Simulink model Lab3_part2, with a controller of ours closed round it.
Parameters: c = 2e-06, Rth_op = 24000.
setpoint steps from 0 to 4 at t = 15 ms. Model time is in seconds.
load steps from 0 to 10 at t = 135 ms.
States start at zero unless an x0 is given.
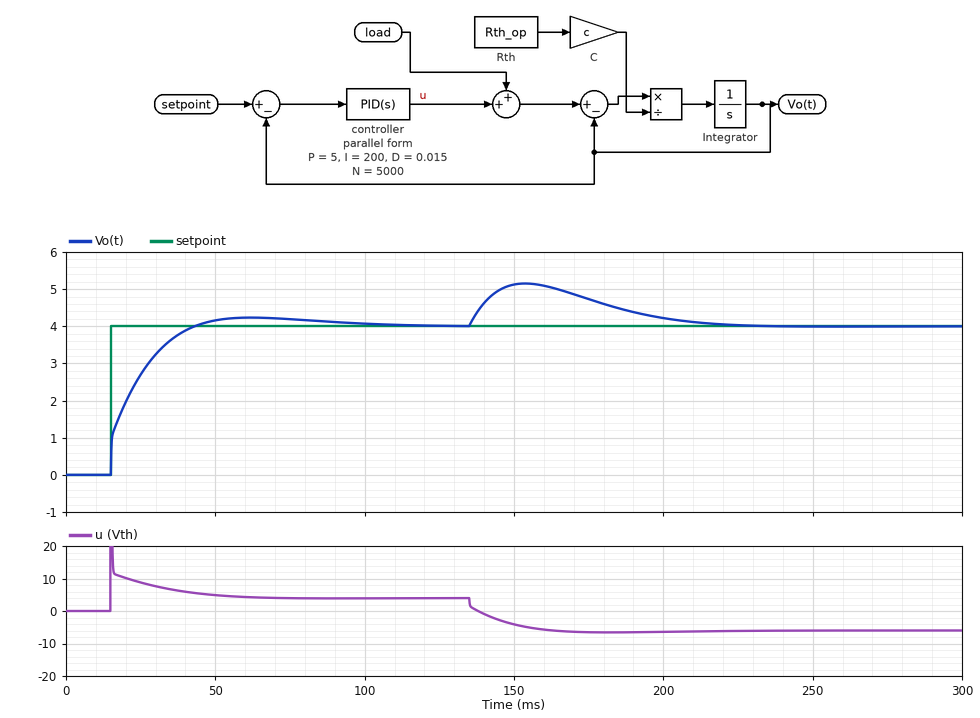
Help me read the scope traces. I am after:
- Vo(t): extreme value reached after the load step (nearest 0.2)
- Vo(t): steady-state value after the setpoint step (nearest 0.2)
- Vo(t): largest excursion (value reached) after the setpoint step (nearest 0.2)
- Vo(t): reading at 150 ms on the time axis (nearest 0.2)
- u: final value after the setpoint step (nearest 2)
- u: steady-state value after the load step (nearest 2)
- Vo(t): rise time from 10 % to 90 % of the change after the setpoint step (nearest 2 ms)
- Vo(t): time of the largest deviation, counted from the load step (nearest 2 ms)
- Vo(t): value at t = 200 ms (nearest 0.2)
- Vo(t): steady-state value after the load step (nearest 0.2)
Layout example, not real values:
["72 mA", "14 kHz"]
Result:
["5.2", "4.0", "4.2", "5.2", "4", "-6", "20 ms", "18 ms", "4.2", "4.0"]
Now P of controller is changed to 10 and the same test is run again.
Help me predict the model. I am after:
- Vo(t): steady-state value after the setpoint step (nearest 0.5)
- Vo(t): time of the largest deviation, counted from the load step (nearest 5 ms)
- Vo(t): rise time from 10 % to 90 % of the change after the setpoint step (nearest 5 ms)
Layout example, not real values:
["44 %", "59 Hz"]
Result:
["4.0", "15 ms", "15 ms"]
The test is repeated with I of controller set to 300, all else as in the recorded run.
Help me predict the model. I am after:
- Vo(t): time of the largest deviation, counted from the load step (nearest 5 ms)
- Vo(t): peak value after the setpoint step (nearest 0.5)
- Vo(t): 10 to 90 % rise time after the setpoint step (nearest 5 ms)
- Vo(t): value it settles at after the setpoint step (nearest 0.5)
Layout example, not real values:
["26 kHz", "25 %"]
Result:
["15 ms", "4.5", "15 ms", "4.0"]
